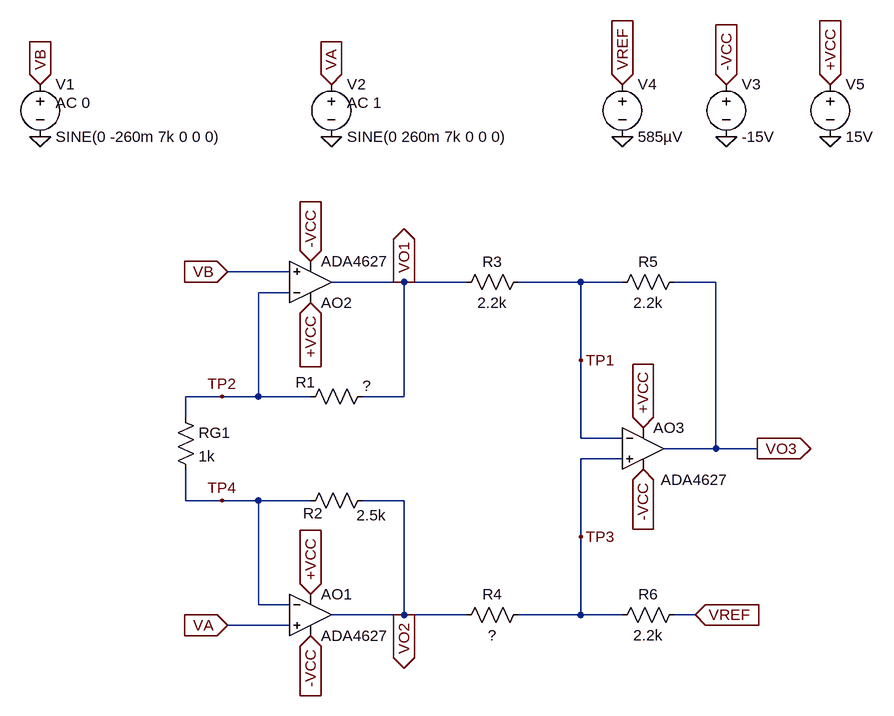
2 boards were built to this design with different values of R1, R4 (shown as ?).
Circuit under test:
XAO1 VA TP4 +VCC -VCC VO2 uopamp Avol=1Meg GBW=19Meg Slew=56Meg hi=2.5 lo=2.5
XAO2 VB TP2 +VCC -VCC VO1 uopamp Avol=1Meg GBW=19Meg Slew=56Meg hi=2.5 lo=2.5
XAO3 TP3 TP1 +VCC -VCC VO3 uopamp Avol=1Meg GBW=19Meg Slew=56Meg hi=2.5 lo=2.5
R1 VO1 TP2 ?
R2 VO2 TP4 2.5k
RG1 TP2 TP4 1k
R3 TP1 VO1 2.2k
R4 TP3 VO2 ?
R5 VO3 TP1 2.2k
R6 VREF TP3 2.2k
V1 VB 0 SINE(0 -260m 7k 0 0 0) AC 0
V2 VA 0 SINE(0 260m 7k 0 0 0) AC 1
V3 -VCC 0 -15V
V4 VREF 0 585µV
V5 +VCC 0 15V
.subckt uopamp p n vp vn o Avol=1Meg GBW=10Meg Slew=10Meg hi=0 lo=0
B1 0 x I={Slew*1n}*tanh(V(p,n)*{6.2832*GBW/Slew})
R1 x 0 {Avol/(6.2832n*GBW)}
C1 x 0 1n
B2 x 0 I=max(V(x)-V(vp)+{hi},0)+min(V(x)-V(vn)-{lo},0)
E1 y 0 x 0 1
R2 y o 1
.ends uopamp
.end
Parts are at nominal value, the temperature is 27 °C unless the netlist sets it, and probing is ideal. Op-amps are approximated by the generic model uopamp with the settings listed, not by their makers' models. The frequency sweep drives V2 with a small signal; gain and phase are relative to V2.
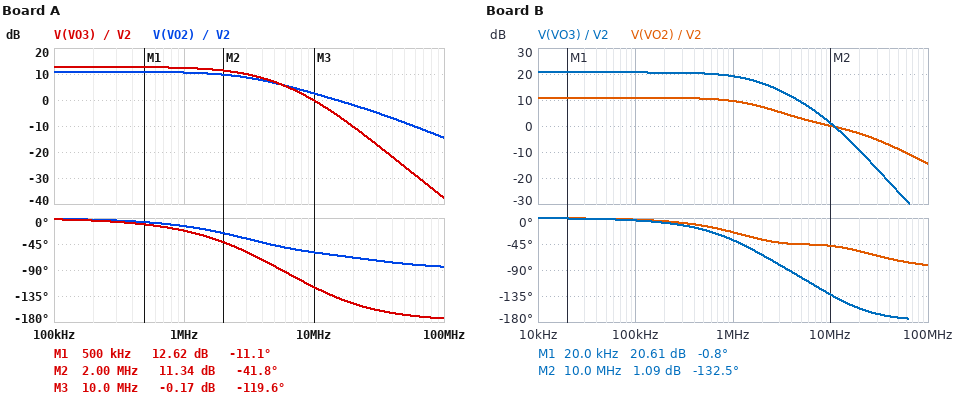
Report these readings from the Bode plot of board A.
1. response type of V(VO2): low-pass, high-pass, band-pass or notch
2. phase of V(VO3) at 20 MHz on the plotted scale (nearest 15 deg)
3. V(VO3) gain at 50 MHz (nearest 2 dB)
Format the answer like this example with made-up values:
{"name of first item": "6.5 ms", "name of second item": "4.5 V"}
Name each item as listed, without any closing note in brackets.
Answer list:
{"response type of V(VO2): low-pass, high-pass, band-pass or notch": "low-pass", "phase of V(VO3) at 20 MHz on the plotted scale": "-150 deg", "V(VO3) gain at 50 MHz": "-26 dB"}
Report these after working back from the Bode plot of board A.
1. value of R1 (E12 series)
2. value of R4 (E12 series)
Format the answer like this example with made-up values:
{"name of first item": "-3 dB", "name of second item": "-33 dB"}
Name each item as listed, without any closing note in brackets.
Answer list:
{"value of R1": "1.8 kΩ", "value of R4": "3.9 kΩ"}
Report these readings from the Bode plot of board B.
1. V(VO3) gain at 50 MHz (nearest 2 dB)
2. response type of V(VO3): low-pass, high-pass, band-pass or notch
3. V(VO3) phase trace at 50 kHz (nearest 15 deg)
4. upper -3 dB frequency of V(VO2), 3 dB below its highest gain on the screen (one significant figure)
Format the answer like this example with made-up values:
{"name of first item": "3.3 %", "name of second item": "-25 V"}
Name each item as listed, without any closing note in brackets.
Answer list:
{"V(VO3) gain at 50 MHz": "-26 dB", "response type of V(VO3): low-pass, high-pass, band-pass or notch": "low-pass", "V(VO3) phase trace at 50 kHz": "0 deg", "upper -3 dB frequency of V(VO2), 3 dB below its highest gain on the screen": "2 MHz"}
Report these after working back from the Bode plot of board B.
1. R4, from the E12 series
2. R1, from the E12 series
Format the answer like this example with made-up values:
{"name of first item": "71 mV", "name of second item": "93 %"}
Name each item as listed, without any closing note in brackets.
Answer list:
{"R4, from the E12 series": "3.9 kΩ", "R1, from the E12 series": "8.2 kΩ"}
